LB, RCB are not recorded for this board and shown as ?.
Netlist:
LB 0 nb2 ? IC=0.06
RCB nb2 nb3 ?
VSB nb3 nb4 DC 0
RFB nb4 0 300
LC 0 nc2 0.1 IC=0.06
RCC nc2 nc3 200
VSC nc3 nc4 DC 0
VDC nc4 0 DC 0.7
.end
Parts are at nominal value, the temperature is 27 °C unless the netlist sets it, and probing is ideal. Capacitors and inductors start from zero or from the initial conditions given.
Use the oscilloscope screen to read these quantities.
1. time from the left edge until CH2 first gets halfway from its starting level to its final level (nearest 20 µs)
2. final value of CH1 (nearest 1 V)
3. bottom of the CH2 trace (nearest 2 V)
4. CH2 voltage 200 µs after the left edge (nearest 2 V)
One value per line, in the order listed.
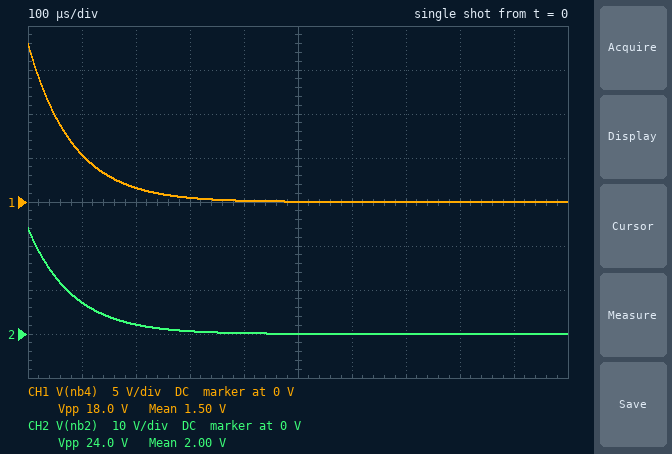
60 µs
0 V
0 V
2 V
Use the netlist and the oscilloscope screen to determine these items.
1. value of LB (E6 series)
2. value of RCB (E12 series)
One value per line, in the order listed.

33 mH
100 Ω
